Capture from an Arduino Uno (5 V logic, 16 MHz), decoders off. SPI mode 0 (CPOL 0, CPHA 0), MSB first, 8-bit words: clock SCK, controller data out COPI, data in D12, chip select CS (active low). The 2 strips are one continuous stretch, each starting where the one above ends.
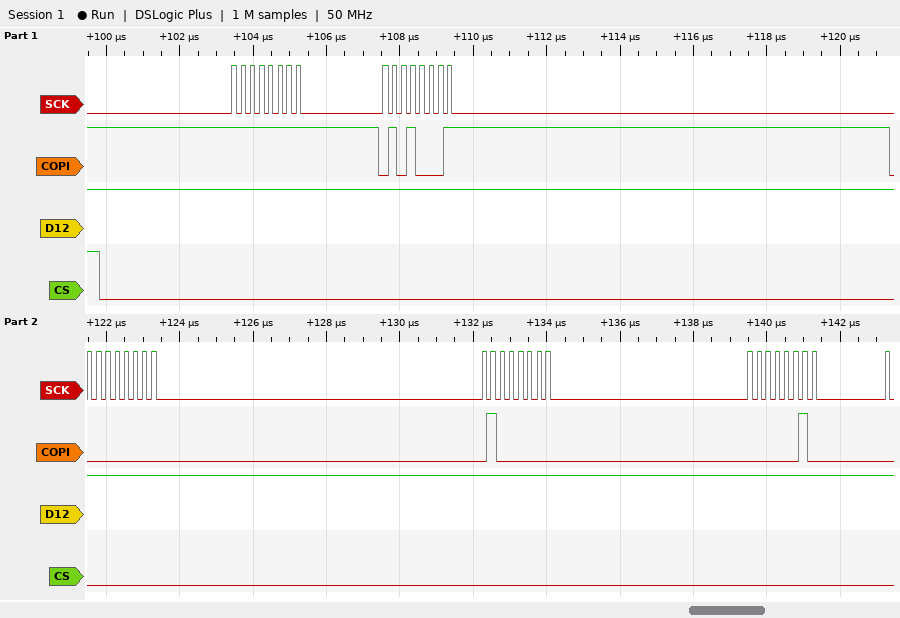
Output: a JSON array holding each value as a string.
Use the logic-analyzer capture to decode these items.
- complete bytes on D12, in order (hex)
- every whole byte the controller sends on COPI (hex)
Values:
["FF FF FF FF FF", "FF 51 00 40 02"]
